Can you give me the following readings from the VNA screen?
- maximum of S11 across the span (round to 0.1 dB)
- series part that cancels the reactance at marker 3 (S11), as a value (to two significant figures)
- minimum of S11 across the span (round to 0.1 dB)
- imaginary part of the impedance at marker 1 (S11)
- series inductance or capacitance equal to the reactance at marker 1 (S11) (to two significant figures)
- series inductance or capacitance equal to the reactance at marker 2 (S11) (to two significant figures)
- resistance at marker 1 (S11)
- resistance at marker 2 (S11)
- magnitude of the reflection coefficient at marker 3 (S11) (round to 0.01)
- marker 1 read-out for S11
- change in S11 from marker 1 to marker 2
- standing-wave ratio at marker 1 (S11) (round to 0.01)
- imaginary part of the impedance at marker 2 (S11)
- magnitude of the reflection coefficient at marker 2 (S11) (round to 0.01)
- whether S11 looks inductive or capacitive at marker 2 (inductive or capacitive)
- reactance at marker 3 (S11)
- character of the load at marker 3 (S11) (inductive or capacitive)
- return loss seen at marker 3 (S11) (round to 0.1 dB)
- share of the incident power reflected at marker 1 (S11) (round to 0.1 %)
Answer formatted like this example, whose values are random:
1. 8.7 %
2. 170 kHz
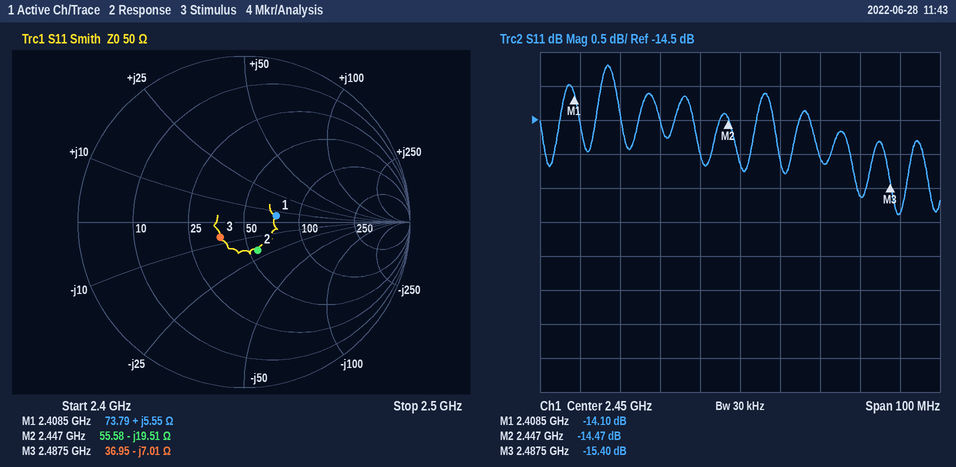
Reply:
1. -13.7 dB
2. 450 pH
3. -15.9 dB
4. +5.55 Ω
5. 370 pH
6. 3.3 pF
7. 73.79 Ω
8. 55.58 Ω
9. 0.17
10. -14.10 dB
11. -0.37 dB
12. 1.49
13. -19.51 Ω
14. 0.19
15. capacitive
16. -7.01 Ω
17. capacitive
18. 15.4 dB
19. 3.9 %
